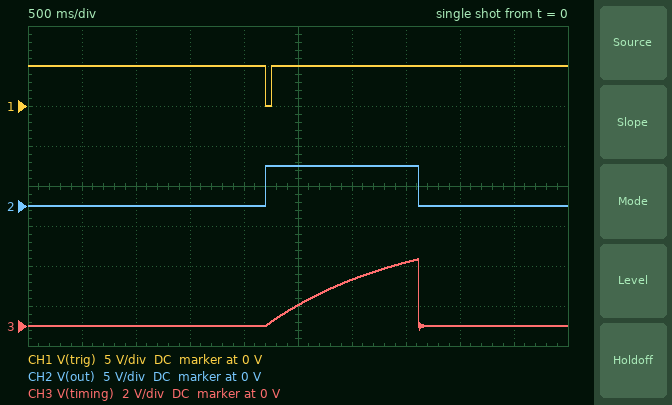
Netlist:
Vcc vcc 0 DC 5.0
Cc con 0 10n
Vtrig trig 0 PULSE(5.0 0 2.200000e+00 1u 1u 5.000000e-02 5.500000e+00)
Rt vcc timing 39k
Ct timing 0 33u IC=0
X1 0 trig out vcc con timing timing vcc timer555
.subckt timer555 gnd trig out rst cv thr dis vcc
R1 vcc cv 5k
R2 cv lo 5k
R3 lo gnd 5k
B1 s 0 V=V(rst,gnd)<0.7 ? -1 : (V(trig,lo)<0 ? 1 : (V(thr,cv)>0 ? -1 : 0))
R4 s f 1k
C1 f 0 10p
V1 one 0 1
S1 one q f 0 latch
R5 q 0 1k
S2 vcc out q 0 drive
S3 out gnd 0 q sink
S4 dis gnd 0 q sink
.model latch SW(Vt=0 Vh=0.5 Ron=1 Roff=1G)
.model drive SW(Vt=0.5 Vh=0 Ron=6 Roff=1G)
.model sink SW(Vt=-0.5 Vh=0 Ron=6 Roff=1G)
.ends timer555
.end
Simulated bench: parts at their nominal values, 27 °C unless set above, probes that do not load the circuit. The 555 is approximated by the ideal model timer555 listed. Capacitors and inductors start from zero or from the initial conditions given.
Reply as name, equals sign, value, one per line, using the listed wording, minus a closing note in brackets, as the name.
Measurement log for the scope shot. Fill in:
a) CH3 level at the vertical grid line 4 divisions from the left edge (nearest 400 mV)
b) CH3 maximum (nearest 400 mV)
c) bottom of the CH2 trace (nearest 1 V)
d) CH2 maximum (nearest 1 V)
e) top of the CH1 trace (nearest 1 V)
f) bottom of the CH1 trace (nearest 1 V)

CH3 level at the vertical grid line 4 divisions from the left edge = 0 V
CH3 maximum = 3.2 V
bottom of the CH2 trace = 0 V
CH2 maximum = 5 V
top of the CH1 trace = 5 V
bottom of the CH1 trace = 0 V
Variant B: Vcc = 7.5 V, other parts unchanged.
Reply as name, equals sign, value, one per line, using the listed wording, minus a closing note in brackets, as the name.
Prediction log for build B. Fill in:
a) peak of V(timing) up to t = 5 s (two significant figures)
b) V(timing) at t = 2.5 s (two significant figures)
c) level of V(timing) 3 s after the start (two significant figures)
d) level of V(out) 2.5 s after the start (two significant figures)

peak of V(timing) up to t = 5 s = 5.0 V
V(timing) at t = 2.5 s = 1.6 V
level of V(timing) 3 s after the start = 3.5 V
level of V(out) 2.5 s after the start = 7.5 V
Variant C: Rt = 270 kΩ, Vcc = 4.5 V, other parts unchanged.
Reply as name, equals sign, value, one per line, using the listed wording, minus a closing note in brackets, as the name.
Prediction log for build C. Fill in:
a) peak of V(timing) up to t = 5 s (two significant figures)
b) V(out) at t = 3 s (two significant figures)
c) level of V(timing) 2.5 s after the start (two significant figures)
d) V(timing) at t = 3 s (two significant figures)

peak of V(timing) up to t = 5 s = 1.2 V
V(out) at t = 3 s = 4.5 V
level of V(timing) 2.5 s after the start = 150 mV
V(timing) at t = 3 s = 390 mV
